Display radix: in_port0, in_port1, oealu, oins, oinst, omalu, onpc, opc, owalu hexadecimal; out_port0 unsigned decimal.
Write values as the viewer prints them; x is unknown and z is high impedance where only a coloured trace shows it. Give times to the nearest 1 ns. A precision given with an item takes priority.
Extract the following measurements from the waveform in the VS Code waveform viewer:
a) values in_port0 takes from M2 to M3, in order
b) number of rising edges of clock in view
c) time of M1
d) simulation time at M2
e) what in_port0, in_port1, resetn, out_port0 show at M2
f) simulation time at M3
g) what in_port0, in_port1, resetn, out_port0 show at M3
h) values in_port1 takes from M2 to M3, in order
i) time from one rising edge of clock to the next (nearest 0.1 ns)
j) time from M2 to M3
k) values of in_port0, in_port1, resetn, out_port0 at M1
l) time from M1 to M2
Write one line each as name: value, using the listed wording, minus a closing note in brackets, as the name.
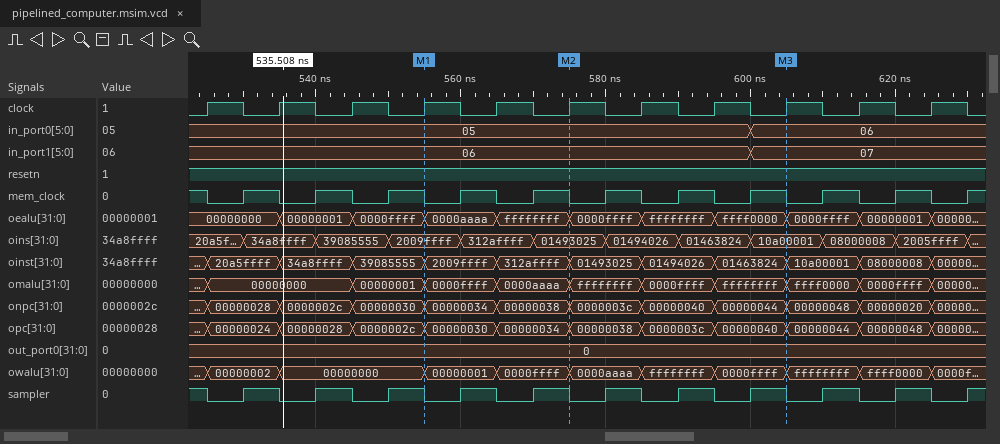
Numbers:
values in_port0 takes from M2 to M3, in order: 05, 06
number of rising edges of clock in view: 11
time of M1: 555 ns
simulation time at M2: 575 ns
what in_port0, in_port1, resetn, out_port0 show at M2: in_port0=05, in_port1=06, resetn=1, out_port0=0
simulation time at M3: 605 ns
what in_port0, in_port1, resetn, out_port0 show at M3: in_port0=06, in_port1=07, resetn=1, out_port0=0
values in_port1 takes from M2 to M3, in order: 06, 07
time from one rising edge of clock to the next: 10 ns
time from M2 to M3: 30 ns
values of in_port0, in_port1, resetn, out_port0 at M1: in_port0=05, in_port1=06, resetn=1, out_port0=0
time from M1 to M2: 20 ns
